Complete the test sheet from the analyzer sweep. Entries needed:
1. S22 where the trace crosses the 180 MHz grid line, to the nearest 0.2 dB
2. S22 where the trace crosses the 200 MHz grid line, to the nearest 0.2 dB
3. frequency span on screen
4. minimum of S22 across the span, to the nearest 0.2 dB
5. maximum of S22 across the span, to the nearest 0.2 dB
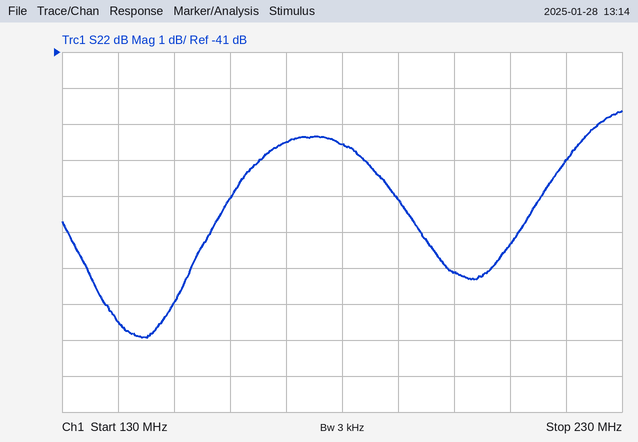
-43.6 dB
-47.2 dB
100 MHz
-49.0 dB
-42.6 dB
